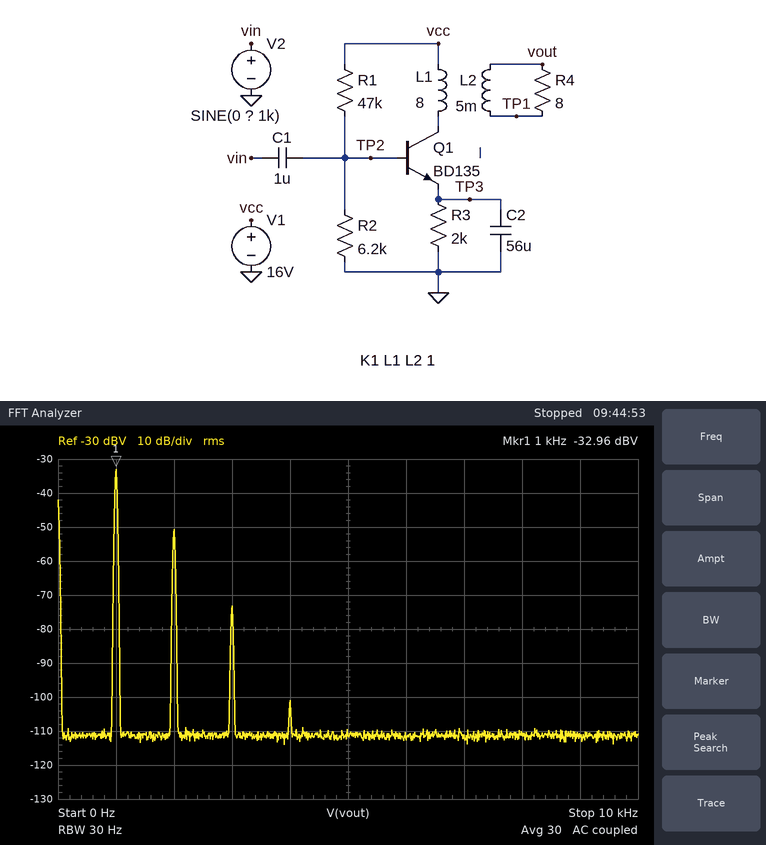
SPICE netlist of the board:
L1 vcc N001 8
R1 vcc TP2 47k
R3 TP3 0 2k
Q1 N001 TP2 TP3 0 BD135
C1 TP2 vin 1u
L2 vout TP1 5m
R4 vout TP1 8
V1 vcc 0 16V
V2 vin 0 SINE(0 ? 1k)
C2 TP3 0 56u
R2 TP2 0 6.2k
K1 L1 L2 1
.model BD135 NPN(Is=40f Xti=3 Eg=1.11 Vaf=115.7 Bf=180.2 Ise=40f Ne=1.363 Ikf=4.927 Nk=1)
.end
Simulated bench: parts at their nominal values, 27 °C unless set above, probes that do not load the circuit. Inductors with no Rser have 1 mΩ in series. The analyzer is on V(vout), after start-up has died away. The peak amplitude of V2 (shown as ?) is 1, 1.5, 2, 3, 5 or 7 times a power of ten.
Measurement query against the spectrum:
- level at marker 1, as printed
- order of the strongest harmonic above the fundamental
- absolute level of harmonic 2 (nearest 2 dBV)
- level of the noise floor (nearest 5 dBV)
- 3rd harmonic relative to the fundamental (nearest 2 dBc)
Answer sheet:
-32.96 dBV
2
-50 dBV
-110 dBV
-40 dBc
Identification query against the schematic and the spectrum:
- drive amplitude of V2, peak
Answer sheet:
15 mV
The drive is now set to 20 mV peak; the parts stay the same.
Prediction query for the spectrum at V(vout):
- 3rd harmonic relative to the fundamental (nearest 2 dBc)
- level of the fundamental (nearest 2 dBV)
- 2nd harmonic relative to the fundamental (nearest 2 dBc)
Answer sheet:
-36 dBc
-30 dBV
-16 dBc
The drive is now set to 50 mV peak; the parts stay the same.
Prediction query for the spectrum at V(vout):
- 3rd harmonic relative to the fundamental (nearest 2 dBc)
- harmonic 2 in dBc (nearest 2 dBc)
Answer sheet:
-20 dBc
-8 dBc
